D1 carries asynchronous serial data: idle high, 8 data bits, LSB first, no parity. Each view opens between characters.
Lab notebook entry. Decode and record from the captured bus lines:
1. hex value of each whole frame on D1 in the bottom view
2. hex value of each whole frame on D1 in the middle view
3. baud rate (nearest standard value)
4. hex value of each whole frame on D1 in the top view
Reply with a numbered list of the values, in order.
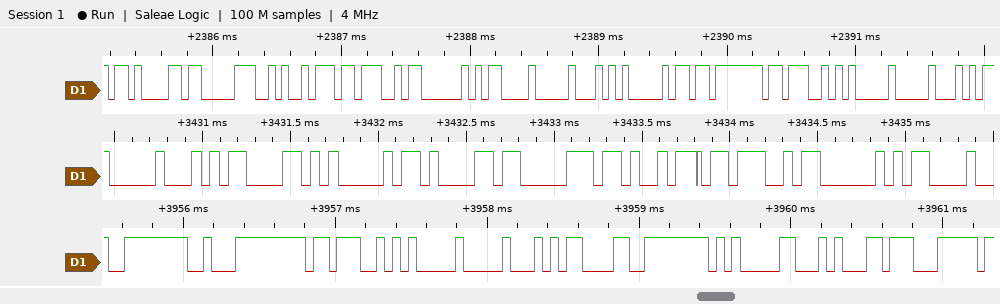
1. FE, E2, 3B, 05, 10, 0D, FE, 05, 14, C7
2. 10, 0D, 05, 0B, 83, 4B, 3B, 03, 0D
3. 19200 baud
4. 0B, 83, 4A, 3B, 03, 0D, 10, 05, DB, 3B, 05, 10
